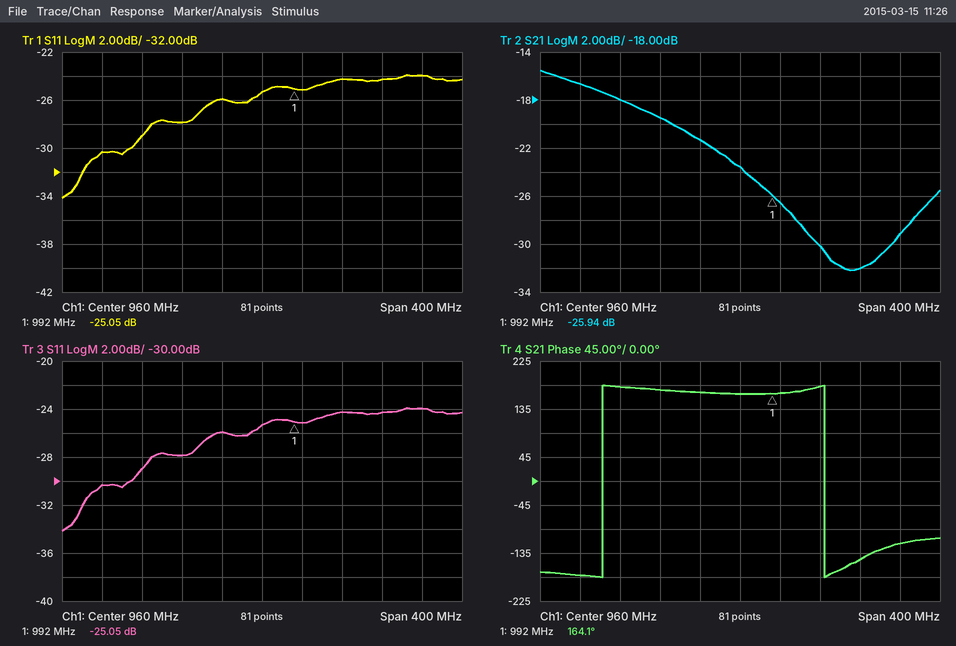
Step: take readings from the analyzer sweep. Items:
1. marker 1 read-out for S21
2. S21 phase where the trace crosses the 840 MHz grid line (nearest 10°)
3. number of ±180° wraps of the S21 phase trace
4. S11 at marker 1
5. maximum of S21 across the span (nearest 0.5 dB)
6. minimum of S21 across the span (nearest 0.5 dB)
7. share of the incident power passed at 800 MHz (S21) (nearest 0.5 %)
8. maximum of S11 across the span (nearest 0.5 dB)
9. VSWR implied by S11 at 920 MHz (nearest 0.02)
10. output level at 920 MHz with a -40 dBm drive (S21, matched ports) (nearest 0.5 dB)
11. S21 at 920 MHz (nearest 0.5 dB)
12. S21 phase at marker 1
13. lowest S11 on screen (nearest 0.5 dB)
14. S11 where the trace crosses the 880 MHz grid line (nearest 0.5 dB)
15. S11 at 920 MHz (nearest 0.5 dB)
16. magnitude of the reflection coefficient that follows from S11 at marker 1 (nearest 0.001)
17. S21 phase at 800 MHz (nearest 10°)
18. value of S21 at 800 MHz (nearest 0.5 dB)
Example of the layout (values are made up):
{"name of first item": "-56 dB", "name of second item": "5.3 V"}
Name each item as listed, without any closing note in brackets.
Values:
{"marker 1 read-out for S21": "-25.94 dB", "S21 phase where the trace crosses the 840 MHz grid line": "180°", "number of ±180° wraps of the S21 phase trace": "2", "S11 at marker 1": "-25.05 dB", "maximum of S21 across the span": "-15.5 dB", "minimum of S21 across the span": "-32.0 dB", "share of the incident power passed at 800 MHz (S21)": "2.0 %", "maximum of S11 across the span": "-24.0 dB", "VSWR implied by S11 at 920 MHz": "1.10", "output level at 920 MHz with a -40 dBm drive (S21, matched ports)": "-61.5 dBm", "S21 at 920 MHz": "-21.5 dB", "S21 phase at marker 1": "164.1°", "lowest S11 on screen": "-34.0 dB", "S11 where the trace crosses the 880 MHz grid line": "-28.0 dB", "S11 at 920 MHz": "-26.0 dB", "magnitude of the reflection coefficient that follows from S11 at marker 1": "0.056", "S21 phase at 800 MHz": "-180°", "value of S21 at 800 MHz": "-16.5 dB"}
